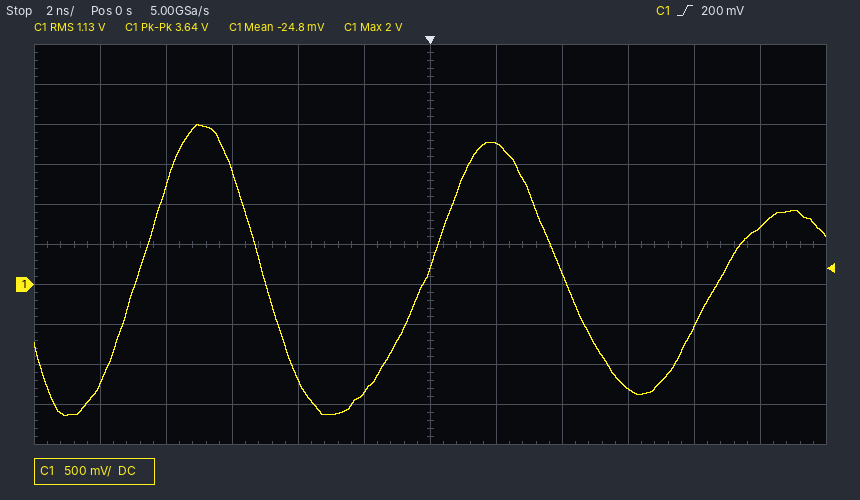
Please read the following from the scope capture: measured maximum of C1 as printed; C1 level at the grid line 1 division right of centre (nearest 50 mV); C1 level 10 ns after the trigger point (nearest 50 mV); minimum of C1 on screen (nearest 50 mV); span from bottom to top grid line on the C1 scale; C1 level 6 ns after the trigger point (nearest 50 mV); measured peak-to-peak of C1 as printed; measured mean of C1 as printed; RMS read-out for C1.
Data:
2 V
1.75 V
700 mV
-1.65 V
5 V
-1.30 V
3.64 V
-24.8 mV
1.13 V
